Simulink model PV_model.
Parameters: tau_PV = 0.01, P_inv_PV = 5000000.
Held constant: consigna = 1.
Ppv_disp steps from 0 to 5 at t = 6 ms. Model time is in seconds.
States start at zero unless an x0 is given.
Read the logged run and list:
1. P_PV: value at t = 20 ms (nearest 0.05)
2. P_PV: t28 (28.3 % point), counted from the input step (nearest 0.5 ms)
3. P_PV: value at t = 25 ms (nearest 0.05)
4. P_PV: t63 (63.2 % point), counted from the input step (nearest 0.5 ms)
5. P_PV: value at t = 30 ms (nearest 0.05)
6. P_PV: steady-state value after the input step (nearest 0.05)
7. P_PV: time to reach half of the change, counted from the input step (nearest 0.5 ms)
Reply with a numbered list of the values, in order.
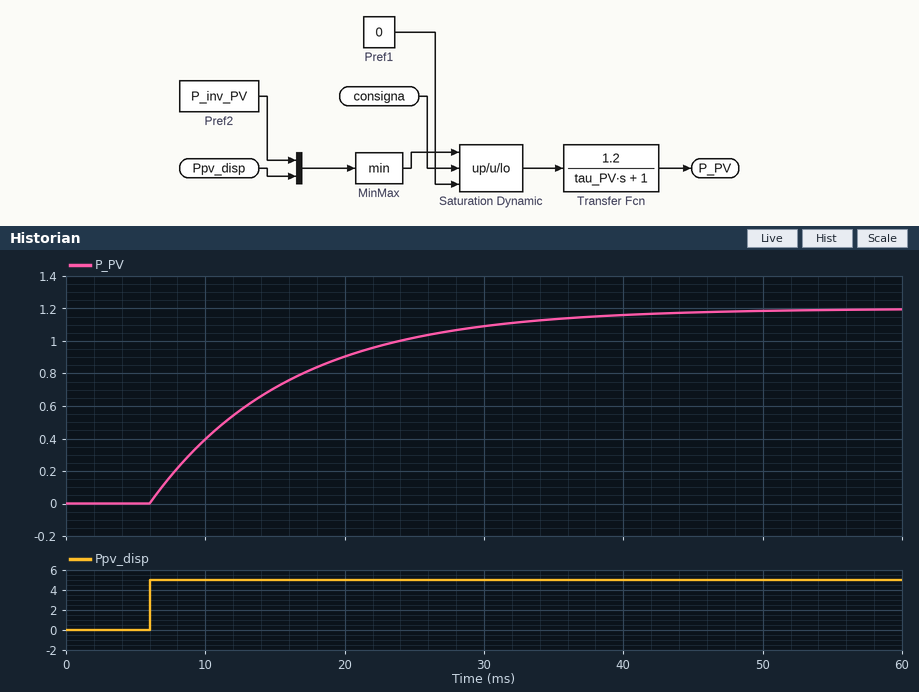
1. 0.90
2. 3.5 ms
3. 1.00
4. 10.0 ms
5. 1.10
6. 1.20
7. 7.0 ms
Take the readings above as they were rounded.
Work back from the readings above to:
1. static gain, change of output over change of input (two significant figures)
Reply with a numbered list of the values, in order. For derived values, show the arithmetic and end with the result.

1. (1.2 - 0) / (5 - 0) = 0.24
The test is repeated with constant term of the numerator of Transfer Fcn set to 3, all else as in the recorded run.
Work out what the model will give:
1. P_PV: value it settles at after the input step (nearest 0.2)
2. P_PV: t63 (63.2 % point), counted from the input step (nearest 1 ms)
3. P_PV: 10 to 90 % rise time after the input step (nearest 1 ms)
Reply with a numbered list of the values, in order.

1. 3.0
2. 10 ms
3. 22 ms
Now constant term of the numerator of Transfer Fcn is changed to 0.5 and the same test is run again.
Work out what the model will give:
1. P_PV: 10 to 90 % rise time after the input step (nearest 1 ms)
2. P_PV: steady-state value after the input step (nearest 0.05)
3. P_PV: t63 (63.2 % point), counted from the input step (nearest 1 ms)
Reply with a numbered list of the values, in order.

1. 22 ms
2. 0.50
3. 10 ms
